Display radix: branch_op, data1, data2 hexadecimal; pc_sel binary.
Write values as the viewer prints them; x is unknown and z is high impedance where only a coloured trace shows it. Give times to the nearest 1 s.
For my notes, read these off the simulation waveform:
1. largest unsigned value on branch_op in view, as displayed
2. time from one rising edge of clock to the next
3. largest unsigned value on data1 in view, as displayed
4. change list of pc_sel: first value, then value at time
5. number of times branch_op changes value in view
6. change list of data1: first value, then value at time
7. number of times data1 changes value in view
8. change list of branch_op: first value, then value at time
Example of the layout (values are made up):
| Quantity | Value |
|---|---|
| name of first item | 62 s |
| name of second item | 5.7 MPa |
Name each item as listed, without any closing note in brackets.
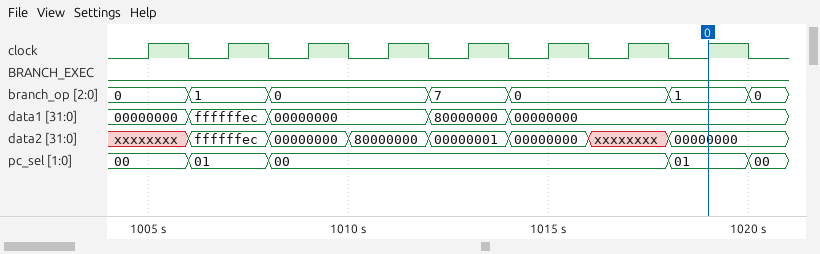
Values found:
| Quantity | Value |
|---|---|
| largest unsigned value on branch_op in view, as displayed | 7 |
| time from one rising edge of clock to the next | 2 s |
| largest unsigned value on data1 in view, as displayed | ffffffec |
| change list of pc_sel: first value, then value at time | 00, 01 at 1006 s, 00 at 1008 s, 01 at 1018 s, 00 at 1020 s |
| number of times branch_op changes value in view | 6 |
| change list of data1: first value, then value at time | 00000000, ffffffec at 1006 s, 00000000 at 1008 s, 80000000 at 1012 s, 00000000 at 1014 s |
| number of times data1 changes value in view | 4 |
| change list of branch_op: first value, then value at time | 0, 1 at 1006 s, 0 at 1008 s, 7 at 1012 s, 0 at 1014 s, 1 at 1018 s, 0 at 1020 s |
